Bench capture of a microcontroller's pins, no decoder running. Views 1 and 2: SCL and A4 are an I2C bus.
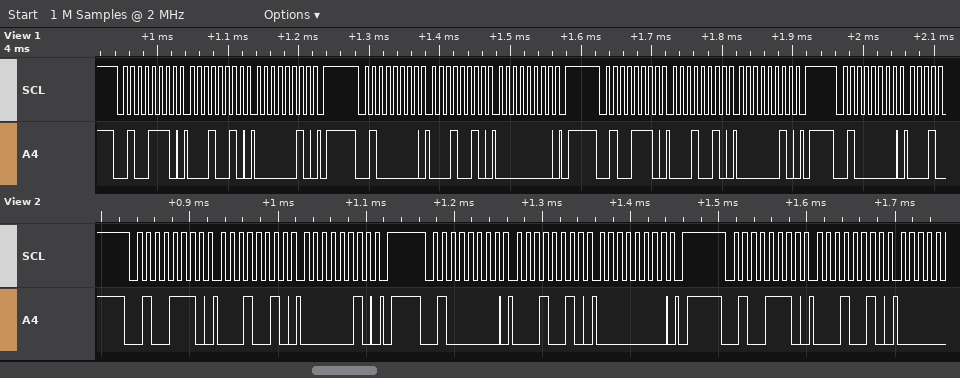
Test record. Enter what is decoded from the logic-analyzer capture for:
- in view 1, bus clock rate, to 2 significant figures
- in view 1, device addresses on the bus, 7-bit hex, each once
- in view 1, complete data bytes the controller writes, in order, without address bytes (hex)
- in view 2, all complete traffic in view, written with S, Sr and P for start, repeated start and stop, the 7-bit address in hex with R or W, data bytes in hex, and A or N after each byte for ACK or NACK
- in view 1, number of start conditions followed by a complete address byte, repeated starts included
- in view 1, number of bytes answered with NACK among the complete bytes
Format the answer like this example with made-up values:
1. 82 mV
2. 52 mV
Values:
1. 100 kHz
2. 0x27 0x20
3. 12 02 12 00 12 02
4. S 27W A 12 A 02 A P S 20W A 12 A 00 A P S 27W A 12 A
5. 4
6. 0
